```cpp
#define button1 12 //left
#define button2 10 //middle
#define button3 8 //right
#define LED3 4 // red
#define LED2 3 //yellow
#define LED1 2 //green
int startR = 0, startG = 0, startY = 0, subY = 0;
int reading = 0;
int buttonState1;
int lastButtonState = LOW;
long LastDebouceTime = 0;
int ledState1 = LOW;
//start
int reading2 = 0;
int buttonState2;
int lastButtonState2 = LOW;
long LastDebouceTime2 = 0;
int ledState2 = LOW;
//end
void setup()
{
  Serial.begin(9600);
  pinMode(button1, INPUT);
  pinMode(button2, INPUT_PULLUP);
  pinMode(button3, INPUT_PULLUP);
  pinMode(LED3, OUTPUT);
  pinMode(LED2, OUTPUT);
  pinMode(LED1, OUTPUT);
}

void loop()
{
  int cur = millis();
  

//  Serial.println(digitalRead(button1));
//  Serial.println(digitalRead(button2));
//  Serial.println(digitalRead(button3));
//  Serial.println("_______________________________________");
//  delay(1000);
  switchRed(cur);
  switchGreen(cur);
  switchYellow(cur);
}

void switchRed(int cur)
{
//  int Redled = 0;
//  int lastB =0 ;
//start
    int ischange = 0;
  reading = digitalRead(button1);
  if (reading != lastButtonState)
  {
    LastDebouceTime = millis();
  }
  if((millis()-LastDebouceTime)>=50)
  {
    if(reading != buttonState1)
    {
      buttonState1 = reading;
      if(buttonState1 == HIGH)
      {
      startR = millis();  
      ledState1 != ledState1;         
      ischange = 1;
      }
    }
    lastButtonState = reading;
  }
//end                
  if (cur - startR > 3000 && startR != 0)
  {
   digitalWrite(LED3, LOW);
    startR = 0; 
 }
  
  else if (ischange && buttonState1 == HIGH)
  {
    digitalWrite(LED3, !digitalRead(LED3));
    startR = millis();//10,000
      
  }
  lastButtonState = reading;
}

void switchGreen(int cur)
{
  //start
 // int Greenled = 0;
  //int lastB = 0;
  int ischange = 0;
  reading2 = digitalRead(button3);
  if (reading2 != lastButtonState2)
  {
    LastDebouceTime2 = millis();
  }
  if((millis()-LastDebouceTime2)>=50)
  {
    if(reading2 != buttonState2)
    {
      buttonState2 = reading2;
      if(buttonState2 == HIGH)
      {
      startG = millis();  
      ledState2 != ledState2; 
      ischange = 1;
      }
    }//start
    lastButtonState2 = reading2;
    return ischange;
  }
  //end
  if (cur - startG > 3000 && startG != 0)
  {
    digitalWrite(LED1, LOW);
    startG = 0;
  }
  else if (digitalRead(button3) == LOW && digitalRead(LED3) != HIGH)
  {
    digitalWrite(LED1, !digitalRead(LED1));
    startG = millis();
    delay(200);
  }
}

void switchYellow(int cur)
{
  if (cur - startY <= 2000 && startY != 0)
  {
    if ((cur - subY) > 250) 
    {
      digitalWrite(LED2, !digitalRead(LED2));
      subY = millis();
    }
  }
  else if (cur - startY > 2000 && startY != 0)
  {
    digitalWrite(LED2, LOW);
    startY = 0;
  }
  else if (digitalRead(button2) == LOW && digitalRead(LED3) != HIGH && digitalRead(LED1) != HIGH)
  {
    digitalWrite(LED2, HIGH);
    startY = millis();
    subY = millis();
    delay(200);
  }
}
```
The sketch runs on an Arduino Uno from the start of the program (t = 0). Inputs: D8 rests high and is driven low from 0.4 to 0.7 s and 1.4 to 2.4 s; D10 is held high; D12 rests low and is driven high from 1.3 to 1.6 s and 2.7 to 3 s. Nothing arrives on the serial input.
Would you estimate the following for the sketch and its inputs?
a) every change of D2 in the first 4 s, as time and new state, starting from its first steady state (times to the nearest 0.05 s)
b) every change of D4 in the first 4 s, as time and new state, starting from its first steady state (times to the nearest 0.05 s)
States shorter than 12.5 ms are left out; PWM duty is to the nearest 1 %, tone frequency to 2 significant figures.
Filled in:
0 s low; 0.4 s high; 3.4 s low
0 s low; 1.35 s high; 2.75 s low
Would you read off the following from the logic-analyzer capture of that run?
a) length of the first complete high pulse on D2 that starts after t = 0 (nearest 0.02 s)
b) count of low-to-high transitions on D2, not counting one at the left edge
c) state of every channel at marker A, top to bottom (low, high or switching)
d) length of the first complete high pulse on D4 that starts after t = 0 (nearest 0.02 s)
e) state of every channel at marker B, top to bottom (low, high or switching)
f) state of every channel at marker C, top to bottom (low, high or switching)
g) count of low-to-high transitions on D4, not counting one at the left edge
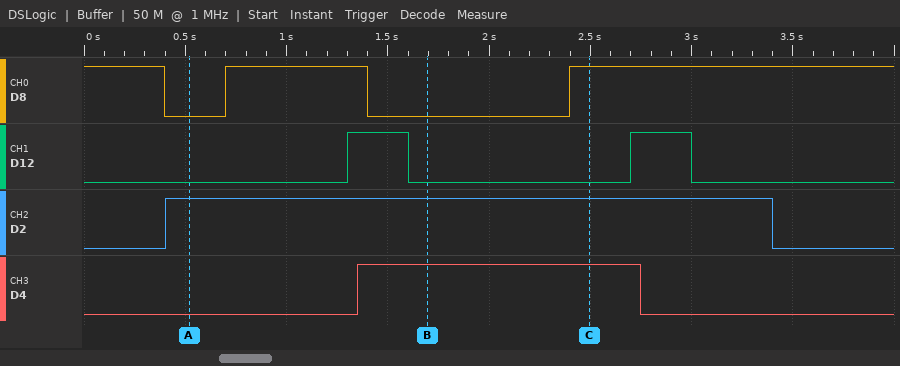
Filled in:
3.00 s
1
D8 low, D12 low, D2 high, D4 low
1.40 s
D8 low, D12 low, D2 high, D4 high
D8 high, D12 low, D2 high, D4 high
1
